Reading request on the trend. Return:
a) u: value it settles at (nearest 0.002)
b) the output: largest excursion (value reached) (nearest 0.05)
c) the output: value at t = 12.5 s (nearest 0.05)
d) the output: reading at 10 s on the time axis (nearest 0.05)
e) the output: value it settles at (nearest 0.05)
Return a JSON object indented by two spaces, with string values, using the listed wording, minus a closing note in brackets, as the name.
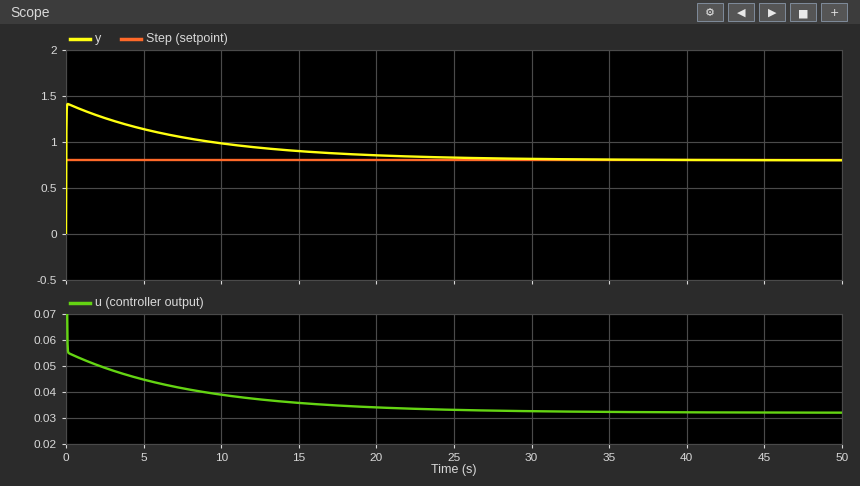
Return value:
{
  "u: value it settles at": "0.032",
  "the output: largest excursion (value reached)": "1.40",
  "the output: value at t = 12.5 s": "0.95",
  "the output: reading at 10 s on the time axis": "1.00",
  "the output: value it settles at": "0.80"
}
